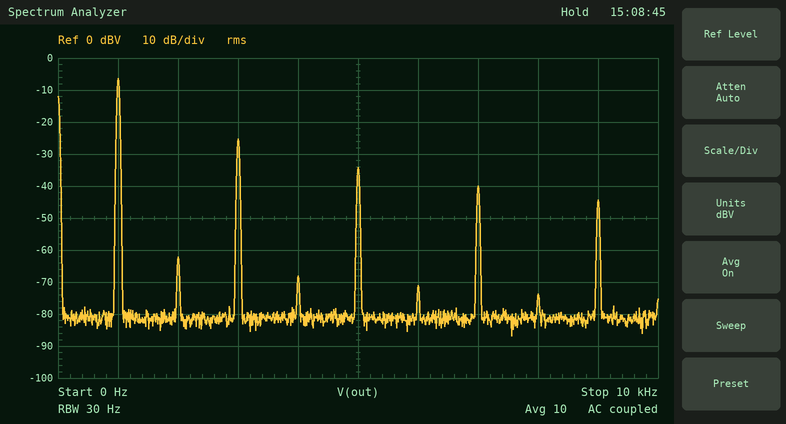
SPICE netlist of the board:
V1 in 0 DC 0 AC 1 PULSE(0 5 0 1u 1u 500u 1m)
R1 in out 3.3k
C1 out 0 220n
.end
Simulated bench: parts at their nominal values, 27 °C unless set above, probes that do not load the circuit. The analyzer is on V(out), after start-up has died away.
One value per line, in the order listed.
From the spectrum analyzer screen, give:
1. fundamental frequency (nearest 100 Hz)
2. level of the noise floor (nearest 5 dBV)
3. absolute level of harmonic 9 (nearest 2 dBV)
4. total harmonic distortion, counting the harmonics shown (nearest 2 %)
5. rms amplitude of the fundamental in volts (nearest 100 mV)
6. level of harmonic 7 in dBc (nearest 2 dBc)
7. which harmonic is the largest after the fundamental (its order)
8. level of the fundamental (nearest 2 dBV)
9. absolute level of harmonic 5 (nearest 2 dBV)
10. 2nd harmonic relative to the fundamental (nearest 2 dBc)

1.0 kHz
-80 dBV
-44 dBV
12 %
500 mV
-34 dBc
3
-6 dBV
-34 dBV
-56 dBc
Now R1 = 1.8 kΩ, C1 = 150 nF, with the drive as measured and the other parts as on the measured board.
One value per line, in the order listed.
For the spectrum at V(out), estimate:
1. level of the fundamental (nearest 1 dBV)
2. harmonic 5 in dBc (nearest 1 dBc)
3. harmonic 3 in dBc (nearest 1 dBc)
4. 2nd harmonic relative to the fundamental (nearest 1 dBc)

1 dBV
-27 dBc
-18 dBc
-55 dBc
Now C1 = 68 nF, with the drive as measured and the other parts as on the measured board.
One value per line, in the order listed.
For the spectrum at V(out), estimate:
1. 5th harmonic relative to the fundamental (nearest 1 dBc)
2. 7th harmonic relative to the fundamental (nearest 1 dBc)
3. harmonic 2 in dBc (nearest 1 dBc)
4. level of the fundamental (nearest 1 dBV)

-26 dBc
-32 dBc
-55 dBc
2 dBV
